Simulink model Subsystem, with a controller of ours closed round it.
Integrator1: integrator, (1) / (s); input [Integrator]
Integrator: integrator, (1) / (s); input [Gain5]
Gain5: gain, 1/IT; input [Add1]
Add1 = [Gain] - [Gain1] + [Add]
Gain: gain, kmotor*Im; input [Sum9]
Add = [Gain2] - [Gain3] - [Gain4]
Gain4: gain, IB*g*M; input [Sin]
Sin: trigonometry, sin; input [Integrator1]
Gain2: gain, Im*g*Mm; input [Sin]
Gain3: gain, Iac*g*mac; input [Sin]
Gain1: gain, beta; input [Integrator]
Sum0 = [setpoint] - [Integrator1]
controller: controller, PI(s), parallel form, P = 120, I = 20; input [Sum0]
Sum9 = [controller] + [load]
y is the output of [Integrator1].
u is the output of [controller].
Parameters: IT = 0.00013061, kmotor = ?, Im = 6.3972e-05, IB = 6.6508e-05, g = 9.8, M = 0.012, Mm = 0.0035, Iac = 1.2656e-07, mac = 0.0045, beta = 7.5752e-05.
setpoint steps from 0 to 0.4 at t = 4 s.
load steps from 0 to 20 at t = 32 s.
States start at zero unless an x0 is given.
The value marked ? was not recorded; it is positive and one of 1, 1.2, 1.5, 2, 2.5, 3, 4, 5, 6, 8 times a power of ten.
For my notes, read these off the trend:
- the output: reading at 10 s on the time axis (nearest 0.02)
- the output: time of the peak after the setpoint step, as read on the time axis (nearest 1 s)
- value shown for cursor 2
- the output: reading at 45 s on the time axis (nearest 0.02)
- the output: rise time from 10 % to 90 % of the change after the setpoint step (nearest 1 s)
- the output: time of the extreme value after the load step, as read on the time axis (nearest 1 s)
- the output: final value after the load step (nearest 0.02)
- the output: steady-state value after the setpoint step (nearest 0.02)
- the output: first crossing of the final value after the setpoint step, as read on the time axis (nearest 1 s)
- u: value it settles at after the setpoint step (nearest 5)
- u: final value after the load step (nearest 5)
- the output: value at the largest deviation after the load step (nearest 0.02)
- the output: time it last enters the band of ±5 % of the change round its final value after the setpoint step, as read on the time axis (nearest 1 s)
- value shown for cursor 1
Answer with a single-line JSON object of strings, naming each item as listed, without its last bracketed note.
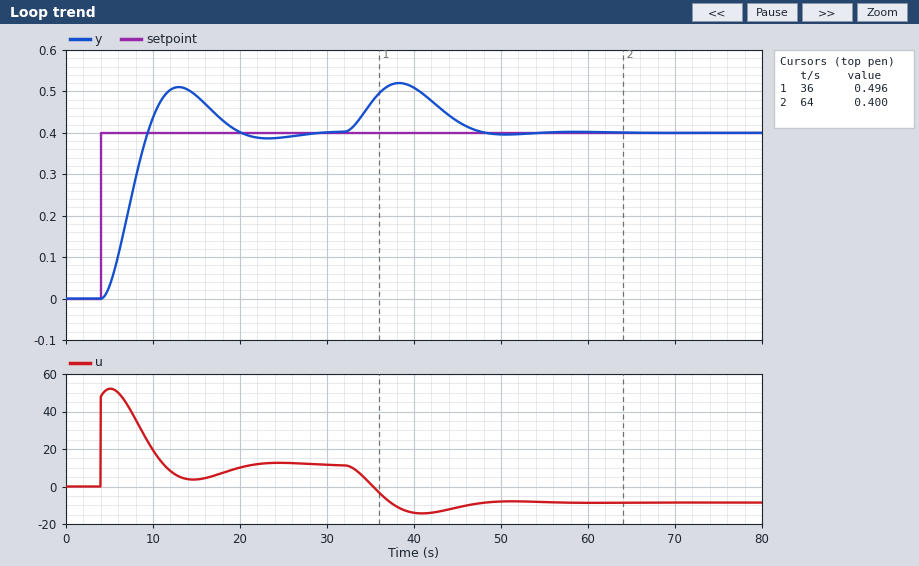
{"the output: reading at 10 s on the time axis": "0.44", "the output: time of the peak after the setpoint step, as read on the time axis": "13 s", "value shown for cursor 2": "0.400", "the output: reading at 45 s on the time axis": "0.42", "the output: rise time from 10 % to 90 % of the change after the setpoint step": "4 s", "the output: time of the extreme value after the load step, as read on the time axis": "38 s", "the output: final value after the load step": "0.40", "the output: steady-state value after the setpoint step": "0.40", "the output: first crossing of the final value after the setpoint step, as read on the time axis": "9 s", "u: value it settles at after the setpoint step": "10", "u: final value after the load step": "-10", "the output: value at the largest deviation after the load step": "0.52", "the output: time it last enters the band of ±5 % of the change round its final value after the setpoint step, as read on the time axis": "19 s", "value shown for cursor 1": "0.496"}
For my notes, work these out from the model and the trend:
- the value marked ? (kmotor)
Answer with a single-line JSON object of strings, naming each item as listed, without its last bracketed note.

{"the value marked ?": "0.003"}
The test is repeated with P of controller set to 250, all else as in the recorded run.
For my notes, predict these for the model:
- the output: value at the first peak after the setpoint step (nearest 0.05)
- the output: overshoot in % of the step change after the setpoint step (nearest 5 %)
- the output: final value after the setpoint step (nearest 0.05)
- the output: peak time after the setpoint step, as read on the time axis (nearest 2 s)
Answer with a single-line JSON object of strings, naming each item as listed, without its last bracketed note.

{"the output: value at the first peak after the setpoint step": "0.50", "the output: overshoot in % of the step change after the setpoint step": "25 %", "the output: final value after the setpoint step": "0.40", "the output: peak time after the setpoint step, as read on the time axis": "10 s"}
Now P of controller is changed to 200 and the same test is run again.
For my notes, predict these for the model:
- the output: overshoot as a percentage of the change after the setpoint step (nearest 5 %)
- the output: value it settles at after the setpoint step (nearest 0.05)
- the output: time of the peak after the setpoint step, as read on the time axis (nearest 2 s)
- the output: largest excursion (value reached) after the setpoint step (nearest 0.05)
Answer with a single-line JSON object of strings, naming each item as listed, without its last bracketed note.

{"the output: overshoot as a percentage of the change after the setpoint step": "25 %", "the output: value it settles at after the setpoint step": "0.40", "the output: time of the peak after the setpoint step, as read on the time axis": "10 s", "the output: largest excursion (value reached) after the setpoint step": "0.50"}
